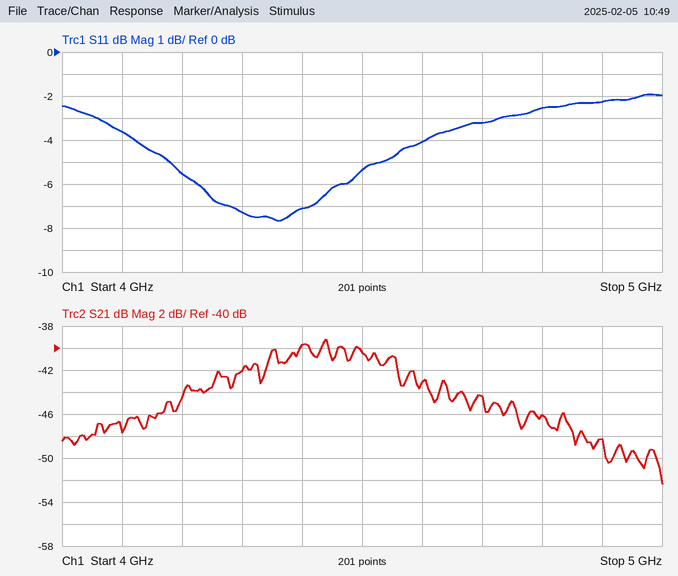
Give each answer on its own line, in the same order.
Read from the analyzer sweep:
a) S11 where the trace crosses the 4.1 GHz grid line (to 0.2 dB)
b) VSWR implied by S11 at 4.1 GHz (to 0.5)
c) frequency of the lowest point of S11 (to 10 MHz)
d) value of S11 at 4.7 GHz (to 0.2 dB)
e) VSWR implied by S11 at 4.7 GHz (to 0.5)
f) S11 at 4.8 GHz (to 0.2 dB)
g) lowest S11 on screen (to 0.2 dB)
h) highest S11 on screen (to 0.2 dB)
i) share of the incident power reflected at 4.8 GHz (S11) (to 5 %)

-3.6 dB
5.0
4.36 GHz
-3.2 dB
5.5
-2.6 dB
-7.6 dB
-2.0 dB
55 %
